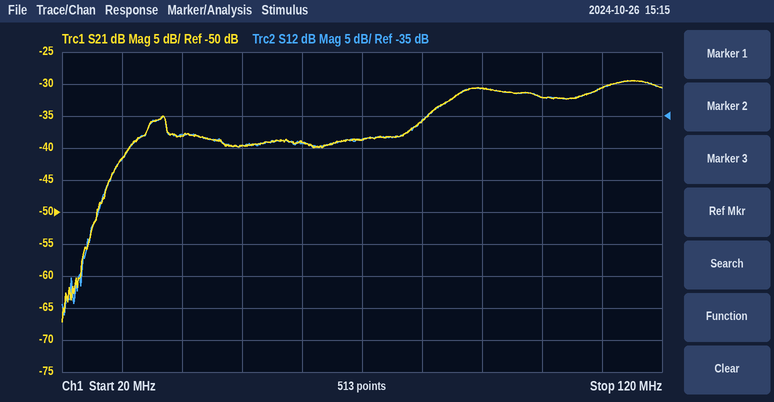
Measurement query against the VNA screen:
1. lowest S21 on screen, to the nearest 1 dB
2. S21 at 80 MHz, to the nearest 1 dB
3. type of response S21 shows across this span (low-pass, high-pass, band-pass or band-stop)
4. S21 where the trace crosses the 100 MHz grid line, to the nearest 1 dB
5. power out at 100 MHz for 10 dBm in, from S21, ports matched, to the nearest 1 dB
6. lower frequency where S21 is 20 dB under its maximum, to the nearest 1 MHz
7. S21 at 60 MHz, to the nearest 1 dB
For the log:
-67 dB
-36 dB
high-pass
-32 dB
-22 dBm
26 MHz
-39 dB
